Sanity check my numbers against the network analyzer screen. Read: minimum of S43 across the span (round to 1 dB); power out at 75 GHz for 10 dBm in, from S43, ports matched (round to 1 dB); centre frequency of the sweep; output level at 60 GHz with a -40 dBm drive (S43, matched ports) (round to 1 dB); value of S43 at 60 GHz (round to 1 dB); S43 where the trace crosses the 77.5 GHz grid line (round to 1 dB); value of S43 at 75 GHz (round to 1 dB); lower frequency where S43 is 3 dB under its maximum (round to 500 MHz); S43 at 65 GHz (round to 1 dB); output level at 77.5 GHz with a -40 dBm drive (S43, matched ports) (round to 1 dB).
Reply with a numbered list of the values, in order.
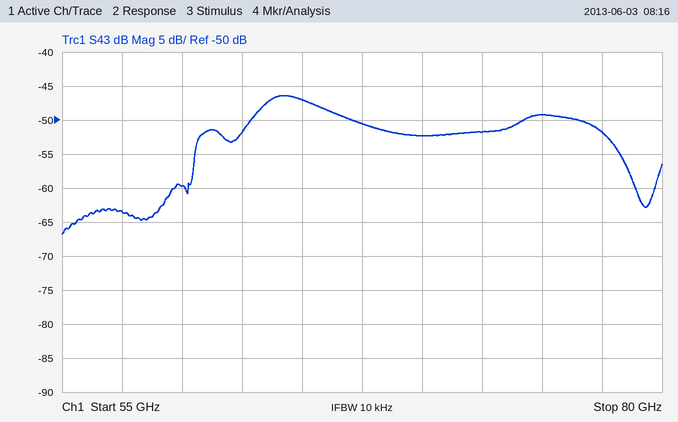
1. -67 dB
2. -39 dBm
3. 67.5 GHz
4. -100 dBm
5. -60 dB
6. -52 dB
7. -49 dB
8. 63.0 GHz
9. -47 dB
10. -92 dBm
